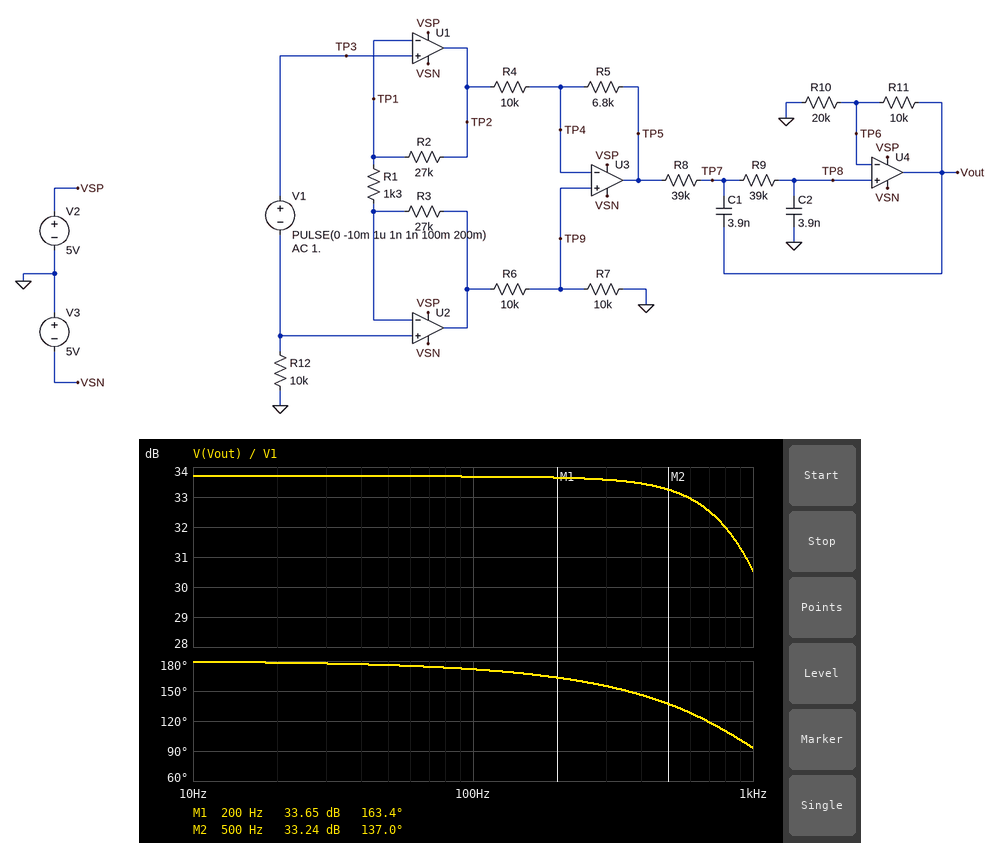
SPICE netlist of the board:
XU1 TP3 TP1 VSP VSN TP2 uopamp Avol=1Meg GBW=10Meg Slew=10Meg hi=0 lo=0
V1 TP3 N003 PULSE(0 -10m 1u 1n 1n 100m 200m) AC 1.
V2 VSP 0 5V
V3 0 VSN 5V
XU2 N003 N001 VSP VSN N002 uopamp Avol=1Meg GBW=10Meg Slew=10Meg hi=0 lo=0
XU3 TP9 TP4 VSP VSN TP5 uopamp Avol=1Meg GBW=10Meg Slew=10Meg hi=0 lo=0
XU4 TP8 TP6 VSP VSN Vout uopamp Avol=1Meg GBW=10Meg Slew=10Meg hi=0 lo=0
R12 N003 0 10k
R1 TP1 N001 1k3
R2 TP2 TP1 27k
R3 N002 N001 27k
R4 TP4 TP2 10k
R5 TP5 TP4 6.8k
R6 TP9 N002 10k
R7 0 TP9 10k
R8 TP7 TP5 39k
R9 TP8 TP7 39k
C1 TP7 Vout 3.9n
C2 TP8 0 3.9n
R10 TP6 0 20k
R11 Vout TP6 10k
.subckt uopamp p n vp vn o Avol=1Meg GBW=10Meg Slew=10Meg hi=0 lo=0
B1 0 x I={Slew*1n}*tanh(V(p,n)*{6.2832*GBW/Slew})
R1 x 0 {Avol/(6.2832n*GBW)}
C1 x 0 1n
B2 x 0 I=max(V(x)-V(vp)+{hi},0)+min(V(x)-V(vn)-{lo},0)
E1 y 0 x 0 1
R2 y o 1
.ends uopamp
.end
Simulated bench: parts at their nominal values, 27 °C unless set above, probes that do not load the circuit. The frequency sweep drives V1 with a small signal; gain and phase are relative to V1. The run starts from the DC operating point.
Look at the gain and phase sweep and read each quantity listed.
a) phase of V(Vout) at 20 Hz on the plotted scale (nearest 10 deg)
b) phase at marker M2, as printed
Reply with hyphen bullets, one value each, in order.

- 180 deg
- 137.0 deg
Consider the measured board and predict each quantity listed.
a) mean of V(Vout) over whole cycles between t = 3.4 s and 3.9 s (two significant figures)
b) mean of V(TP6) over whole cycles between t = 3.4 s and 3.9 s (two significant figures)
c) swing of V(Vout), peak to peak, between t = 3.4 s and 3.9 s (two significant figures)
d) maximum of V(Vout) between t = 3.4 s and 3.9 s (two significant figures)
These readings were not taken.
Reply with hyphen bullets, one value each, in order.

- 240 mV
- 160 mV
- 520 mV
- 500 mV
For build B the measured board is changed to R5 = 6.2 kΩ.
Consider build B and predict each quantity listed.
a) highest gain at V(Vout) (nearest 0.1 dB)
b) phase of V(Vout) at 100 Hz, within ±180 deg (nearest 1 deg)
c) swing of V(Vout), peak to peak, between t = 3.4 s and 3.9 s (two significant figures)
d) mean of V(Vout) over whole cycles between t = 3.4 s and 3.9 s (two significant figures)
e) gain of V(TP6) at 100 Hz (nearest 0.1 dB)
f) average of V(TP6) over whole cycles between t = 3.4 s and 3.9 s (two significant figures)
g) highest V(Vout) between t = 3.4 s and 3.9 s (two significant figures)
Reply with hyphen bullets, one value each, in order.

- 33.2 dB
- 172 deg
- 490 mV
- 230 mV
- 29.6 dB
- 150 mV
- 470 mV
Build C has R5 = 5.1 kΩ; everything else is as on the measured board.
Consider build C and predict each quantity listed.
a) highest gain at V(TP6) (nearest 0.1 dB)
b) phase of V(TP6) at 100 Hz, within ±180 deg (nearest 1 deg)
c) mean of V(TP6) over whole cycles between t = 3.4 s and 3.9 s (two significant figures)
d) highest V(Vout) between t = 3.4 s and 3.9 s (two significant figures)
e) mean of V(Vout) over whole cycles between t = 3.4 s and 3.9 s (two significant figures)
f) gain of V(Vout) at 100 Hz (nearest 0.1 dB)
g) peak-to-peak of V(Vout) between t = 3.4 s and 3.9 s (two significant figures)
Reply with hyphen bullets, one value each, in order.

- 28.6 dB
- 172 deg
- 130 mV
- 420 mV
- 200 mV
- 32.1 dB
- 430 mV
